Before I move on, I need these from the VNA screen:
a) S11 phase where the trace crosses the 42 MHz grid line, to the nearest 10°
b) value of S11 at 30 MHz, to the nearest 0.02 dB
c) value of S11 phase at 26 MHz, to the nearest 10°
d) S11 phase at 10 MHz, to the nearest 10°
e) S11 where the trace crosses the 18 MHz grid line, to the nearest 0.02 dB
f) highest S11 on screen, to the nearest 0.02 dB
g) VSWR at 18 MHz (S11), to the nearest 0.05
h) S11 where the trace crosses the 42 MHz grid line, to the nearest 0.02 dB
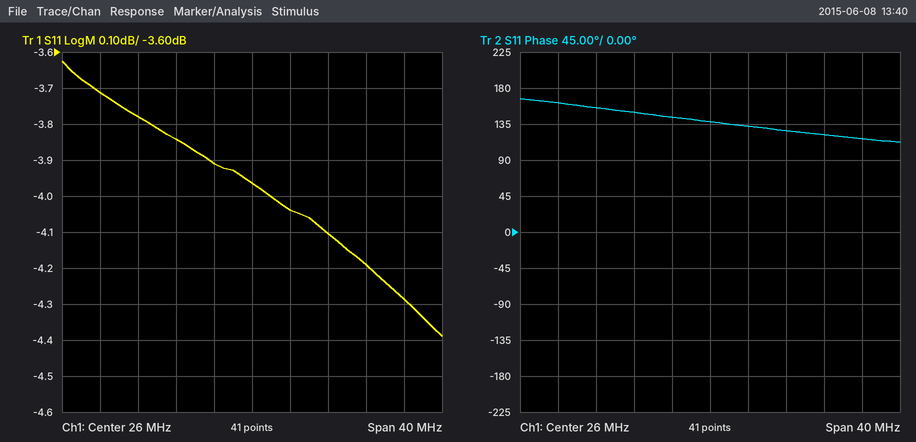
120°
-4.04 dB
140°
160°
-3.84 dB
-3.62 dB
4.60
-4.28 dB
